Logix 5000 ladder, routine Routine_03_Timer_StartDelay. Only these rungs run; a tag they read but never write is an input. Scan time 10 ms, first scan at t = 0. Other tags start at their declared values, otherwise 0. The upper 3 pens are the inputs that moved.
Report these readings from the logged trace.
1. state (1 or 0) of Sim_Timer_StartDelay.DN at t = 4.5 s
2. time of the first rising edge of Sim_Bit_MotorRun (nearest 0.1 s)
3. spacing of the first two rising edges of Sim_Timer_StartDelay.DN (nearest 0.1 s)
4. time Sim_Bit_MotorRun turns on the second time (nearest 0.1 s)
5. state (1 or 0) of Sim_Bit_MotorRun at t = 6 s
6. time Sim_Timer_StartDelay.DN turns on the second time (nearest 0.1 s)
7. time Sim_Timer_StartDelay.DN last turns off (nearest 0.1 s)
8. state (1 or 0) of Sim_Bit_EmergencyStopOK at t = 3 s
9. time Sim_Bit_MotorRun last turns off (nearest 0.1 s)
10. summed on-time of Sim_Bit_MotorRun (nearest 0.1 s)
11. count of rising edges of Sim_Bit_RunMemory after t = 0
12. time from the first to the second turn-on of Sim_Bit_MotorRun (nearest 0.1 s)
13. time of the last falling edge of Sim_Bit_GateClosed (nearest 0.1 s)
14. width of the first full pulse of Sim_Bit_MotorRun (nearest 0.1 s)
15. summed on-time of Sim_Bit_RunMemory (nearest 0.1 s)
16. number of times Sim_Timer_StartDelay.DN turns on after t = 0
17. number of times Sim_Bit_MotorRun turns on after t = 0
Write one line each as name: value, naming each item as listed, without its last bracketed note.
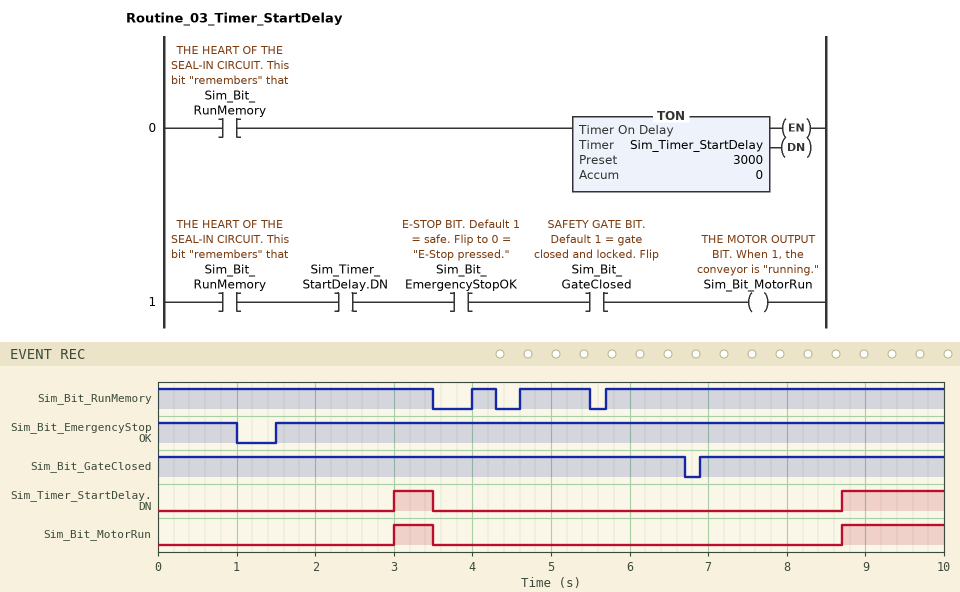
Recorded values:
state (1 or 0) of Sim_Timer_StartDelay.DN at t = 4.5 s: 0
time of the first rising edge of Sim_Bit_MotorRun: 3.0 s
spacing of the first two rising edges of Sim_Timer_StartDelay.DN: 5.7 s
time Sim_Bit_MotorRun turns on the second time: 8.7 s
state (1 or 0) of Sim_Bit_MotorRun at t = 6 s: 0
time Sim_Timer_StartDelay.DN turns on the second time: 8.7 s
time Sim_Timer_StartDelay.DN last turns off: 3.5 s
state (1 or 0) of Sim_Bit_EmergencyStopOK at t = 3 s: 1
time Sim_Bit_MotorRun last turns off: 3.5 s
summed on-time of Sim_Bit_MotorRun: 1.8 s
count of rising edges of Sim_Bit_RunMemory after t = 0: 3
time from the first to the second turn-on of Sim_Bit_MotorRun: 5.7 s
time of the last falling edge of Sim_Bit_GateClosed: 6.7 s
width of the first full pulse of Sim_Bit_MotorRun: 0.5 s
summed on-time of Sim_Bit_RunMemory: 9.0 s
number of times Sim_Timer_StartDelay.DN turns on after t = 0: 2
number of times Sim_Bit_MotorRun turns on after t = 0: 2
